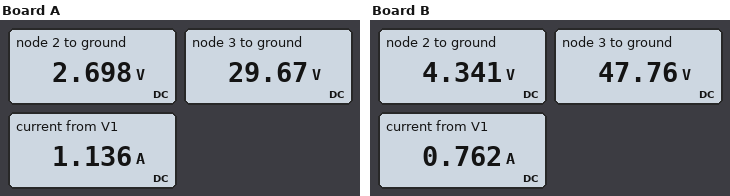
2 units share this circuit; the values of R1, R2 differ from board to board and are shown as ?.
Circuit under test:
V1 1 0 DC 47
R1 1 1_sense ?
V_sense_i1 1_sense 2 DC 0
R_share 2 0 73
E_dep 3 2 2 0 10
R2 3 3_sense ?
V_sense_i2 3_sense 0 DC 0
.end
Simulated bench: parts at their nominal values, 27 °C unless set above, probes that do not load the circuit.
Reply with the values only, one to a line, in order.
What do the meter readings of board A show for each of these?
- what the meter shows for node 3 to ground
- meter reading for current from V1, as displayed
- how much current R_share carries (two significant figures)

29.67 V
1.136 A
37 mA
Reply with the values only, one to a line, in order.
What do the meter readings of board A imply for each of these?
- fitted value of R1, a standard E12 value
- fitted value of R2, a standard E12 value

39 Ω
27 Ω
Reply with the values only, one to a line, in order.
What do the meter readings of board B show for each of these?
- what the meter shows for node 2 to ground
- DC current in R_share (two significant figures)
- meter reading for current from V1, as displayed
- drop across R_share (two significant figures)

4.341 V
59 mA
0.762 A
4.3 V
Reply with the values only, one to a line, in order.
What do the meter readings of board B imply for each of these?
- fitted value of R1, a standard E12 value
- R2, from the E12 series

56 Ω
68 Ω
